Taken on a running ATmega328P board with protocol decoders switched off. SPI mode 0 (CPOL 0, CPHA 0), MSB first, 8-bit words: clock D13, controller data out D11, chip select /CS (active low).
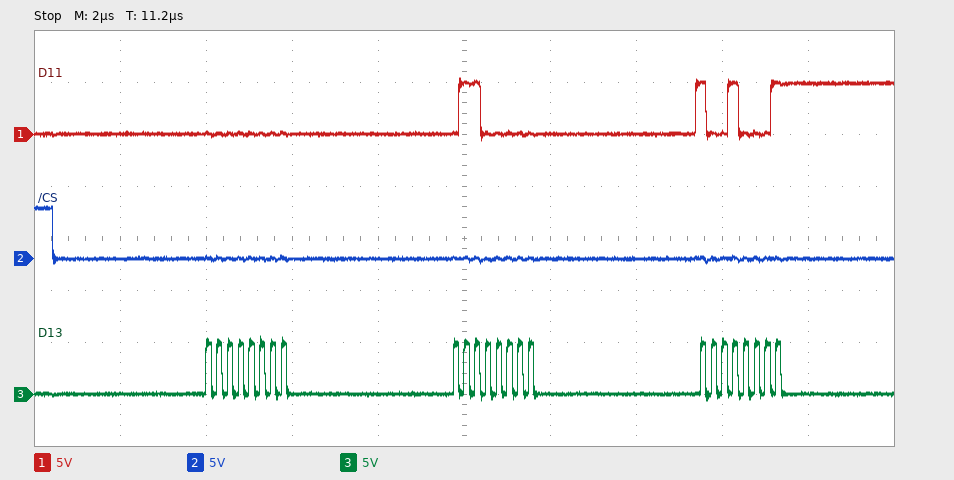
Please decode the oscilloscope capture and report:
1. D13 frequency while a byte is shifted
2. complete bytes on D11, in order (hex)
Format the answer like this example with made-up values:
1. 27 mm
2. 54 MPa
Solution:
1. 4 MHz
2. 0x00 0x60 0x91
